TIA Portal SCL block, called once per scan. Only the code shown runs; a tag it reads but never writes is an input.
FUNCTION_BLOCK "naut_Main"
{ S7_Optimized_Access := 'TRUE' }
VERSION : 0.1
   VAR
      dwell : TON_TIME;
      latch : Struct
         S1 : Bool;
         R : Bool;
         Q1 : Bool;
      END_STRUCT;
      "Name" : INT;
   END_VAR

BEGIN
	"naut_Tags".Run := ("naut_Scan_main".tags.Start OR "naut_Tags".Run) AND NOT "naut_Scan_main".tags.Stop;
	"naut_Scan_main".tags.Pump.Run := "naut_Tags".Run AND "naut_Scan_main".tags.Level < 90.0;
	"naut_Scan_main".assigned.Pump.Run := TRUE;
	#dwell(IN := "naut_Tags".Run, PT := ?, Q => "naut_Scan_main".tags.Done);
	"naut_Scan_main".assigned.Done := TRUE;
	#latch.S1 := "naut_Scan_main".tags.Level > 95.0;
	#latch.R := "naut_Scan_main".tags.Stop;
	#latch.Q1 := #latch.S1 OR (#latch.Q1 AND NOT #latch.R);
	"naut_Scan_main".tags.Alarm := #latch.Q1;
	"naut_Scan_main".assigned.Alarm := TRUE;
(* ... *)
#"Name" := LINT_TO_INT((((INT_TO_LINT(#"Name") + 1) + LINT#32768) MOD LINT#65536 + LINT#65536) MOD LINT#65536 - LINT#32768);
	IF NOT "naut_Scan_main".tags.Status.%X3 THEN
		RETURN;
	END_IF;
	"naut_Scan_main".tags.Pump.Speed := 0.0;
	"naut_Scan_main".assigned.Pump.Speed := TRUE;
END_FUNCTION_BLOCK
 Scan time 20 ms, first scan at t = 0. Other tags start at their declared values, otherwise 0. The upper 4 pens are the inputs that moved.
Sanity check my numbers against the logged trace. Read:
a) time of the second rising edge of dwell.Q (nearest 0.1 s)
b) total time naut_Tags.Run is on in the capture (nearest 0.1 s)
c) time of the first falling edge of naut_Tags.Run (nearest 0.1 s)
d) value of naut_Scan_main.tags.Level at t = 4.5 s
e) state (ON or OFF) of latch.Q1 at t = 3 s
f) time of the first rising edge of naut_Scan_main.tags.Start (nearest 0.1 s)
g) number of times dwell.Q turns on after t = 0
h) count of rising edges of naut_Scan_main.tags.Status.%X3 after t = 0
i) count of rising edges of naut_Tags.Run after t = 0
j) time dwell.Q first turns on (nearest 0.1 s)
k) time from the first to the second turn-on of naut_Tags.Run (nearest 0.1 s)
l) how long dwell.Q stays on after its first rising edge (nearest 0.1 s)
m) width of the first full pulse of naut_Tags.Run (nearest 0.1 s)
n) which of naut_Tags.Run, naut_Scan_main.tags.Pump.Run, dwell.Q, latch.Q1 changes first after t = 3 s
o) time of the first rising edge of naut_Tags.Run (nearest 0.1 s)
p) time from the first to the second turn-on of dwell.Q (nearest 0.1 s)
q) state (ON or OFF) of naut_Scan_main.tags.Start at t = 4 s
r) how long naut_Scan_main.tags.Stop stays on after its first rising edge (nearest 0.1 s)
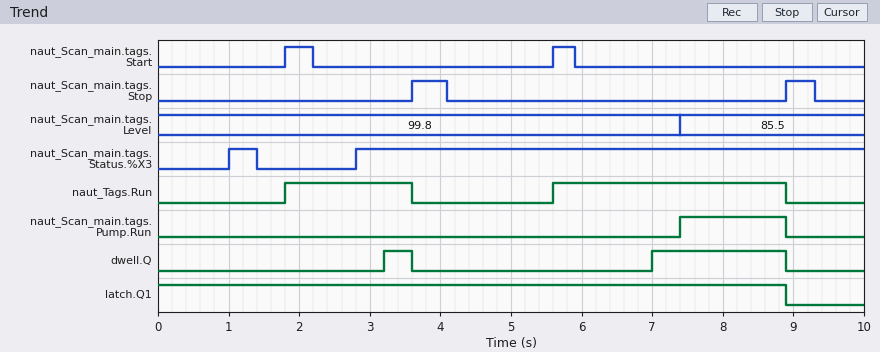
7.0 s
5.1 s
3.6 s
99.8
ON
1.8 s
2
2
2
3.2 s
3.8 s
0.4 s
1.8 s
dwell.Q
1.8 s
3.8 s
OFF
0.5 s
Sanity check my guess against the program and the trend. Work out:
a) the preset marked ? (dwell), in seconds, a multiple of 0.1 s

1.4 s
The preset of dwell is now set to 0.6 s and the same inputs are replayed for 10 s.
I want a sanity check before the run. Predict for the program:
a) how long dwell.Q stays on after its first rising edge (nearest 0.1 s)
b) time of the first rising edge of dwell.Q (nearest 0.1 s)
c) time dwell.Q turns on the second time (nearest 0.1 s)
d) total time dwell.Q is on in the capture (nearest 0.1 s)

1.2 s
2.4 s
6.2 s
3.9 s
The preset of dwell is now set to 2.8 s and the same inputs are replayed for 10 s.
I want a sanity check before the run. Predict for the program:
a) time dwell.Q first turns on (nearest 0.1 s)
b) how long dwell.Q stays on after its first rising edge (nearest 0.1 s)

8.4 s
0.5 s
